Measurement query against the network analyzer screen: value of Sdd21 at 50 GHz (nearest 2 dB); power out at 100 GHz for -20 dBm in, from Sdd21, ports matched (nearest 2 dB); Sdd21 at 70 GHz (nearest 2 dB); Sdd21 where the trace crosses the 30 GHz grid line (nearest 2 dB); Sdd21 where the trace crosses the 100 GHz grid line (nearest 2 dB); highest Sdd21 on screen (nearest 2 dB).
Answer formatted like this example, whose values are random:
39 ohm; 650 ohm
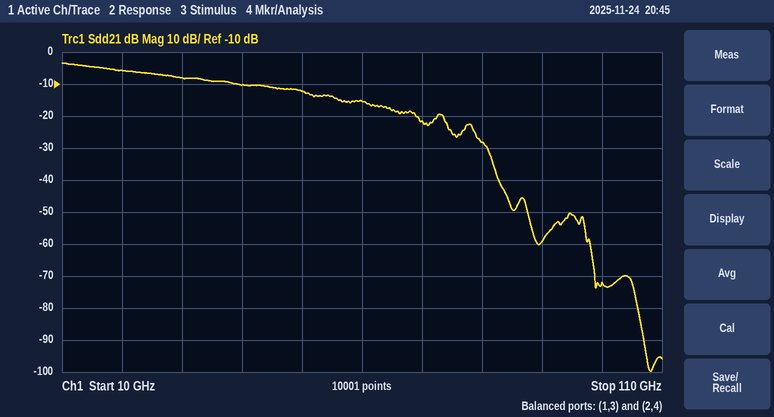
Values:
-12 dB; -92 dBm; -22 dB; -8 dB; -72 dB; -4 dB
